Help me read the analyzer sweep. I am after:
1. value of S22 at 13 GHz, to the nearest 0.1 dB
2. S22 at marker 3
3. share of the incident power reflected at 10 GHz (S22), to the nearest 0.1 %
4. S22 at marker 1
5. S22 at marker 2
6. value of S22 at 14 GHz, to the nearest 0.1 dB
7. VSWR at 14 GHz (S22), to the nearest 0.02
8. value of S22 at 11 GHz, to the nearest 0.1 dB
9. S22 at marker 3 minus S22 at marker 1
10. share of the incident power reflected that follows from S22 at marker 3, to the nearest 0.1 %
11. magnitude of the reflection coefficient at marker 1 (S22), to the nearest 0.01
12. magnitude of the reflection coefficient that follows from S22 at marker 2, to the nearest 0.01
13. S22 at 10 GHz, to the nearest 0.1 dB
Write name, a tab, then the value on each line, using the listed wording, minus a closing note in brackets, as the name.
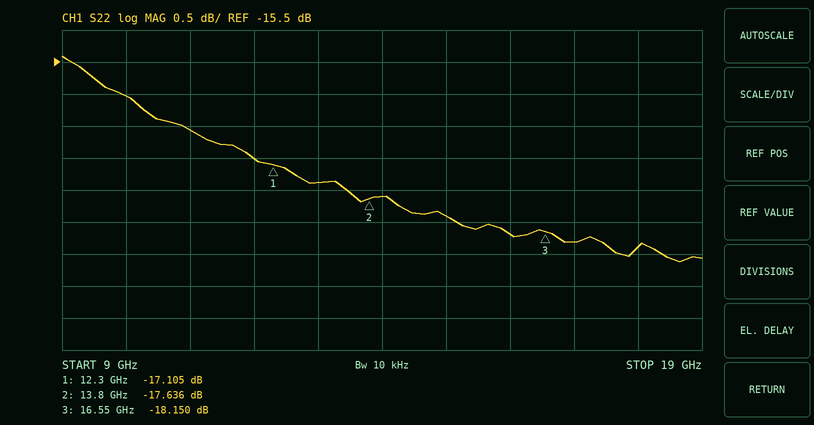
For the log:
value of S22 at 13 GHz, to the nearest 0.1 dB	-17.4 dB
S22 at marker 3	-18.150 dB
share of the incident power reflected at 10 GHz (S22), to the nearest 0.1 %	2.5 %
S22 at marker 1	-17.105 dB
S22 at marker 2	-17.636 dB
value of S22 at 14 GHz, to the nearest 0.1 dB	-17.6 dB
VSWR at 14 GHz (S22), to the nearest 0.02	1.30
value of S22 at 11 GHz, to the nearest 0.1 dB	-16.6 dB
S22 at marker 3 minus S22 at marker 1	-1.045 dB
share of the incident power reflected that follows from S22 at marker 3, to the nearest 0.1 %	1.5 %
magnitude of the reflection coefficient at marker 1 (S22), to the nearest 0.01	0.14
magnitude of the reflection coefficient that follows from S22 at marker 2, to the nearest 0.01	0.13
S22 at 10 GHz, to the nearest 0.1 dB	-16.0 dB
